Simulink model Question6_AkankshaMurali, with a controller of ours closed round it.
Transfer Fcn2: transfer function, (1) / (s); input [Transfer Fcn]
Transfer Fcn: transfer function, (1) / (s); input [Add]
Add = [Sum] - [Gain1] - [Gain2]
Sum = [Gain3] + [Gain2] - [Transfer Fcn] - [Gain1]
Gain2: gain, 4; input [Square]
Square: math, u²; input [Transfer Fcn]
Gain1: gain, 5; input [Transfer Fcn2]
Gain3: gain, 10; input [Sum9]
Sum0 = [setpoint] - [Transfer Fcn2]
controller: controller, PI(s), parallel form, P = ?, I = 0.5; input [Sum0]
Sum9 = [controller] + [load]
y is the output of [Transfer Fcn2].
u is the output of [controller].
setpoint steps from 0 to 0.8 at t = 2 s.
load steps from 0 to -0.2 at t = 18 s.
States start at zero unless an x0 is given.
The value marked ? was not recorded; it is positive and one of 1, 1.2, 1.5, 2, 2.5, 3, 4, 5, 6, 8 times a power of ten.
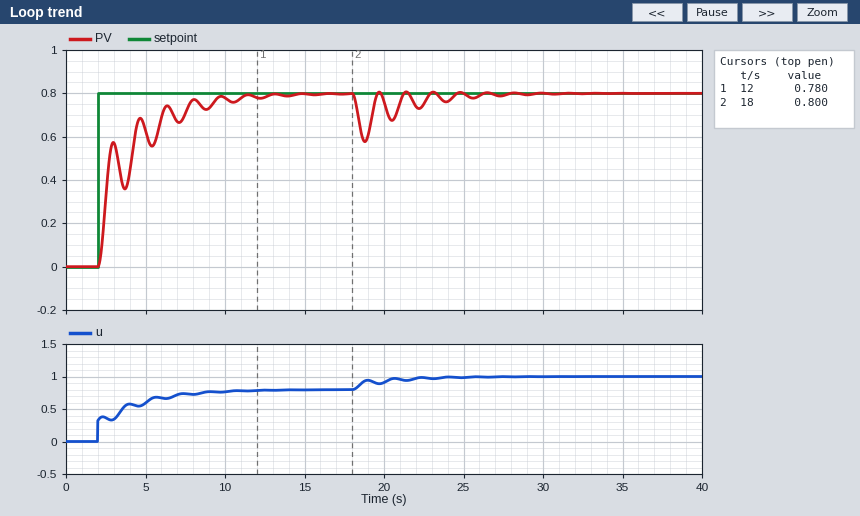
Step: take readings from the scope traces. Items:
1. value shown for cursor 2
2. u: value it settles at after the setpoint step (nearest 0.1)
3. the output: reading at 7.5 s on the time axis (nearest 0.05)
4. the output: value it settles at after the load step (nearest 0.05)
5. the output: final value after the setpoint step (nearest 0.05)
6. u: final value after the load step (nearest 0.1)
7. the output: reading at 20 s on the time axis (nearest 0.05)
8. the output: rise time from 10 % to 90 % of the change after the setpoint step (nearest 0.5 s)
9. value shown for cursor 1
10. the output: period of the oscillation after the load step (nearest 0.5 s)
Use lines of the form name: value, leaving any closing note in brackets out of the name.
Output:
value shown for cursor 2: 0.800
u: value it settles at after the setpoint step: 0.8
the output: reading at 7.5 s on the time axis: 0.70
the output: value it settles at after the load step: 0.80
the output: final value after the setpoint step: 0.80
u: final value after the load step: 1.0
the output: reading at 20 s on the time axis: 0.75
the output: rise time from 10 % to 90 % of the change after the setpoint step: 4.0 s
value shown for cursor 1: 0.780
the output: period of the oscillation after the load step: 1.5 s
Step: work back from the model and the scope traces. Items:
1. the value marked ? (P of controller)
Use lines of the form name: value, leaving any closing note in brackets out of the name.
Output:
the value marked ?: 0.4
